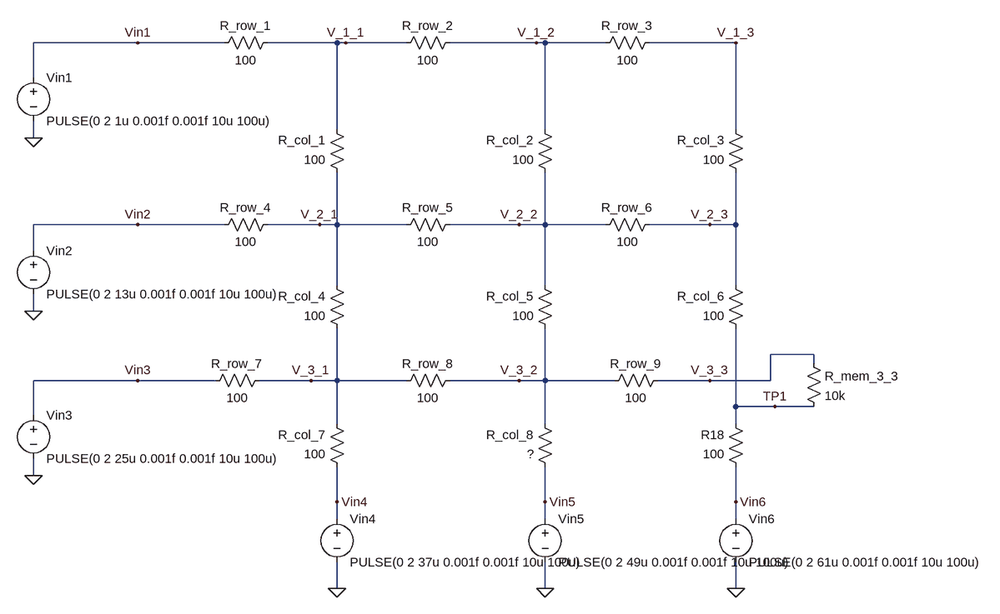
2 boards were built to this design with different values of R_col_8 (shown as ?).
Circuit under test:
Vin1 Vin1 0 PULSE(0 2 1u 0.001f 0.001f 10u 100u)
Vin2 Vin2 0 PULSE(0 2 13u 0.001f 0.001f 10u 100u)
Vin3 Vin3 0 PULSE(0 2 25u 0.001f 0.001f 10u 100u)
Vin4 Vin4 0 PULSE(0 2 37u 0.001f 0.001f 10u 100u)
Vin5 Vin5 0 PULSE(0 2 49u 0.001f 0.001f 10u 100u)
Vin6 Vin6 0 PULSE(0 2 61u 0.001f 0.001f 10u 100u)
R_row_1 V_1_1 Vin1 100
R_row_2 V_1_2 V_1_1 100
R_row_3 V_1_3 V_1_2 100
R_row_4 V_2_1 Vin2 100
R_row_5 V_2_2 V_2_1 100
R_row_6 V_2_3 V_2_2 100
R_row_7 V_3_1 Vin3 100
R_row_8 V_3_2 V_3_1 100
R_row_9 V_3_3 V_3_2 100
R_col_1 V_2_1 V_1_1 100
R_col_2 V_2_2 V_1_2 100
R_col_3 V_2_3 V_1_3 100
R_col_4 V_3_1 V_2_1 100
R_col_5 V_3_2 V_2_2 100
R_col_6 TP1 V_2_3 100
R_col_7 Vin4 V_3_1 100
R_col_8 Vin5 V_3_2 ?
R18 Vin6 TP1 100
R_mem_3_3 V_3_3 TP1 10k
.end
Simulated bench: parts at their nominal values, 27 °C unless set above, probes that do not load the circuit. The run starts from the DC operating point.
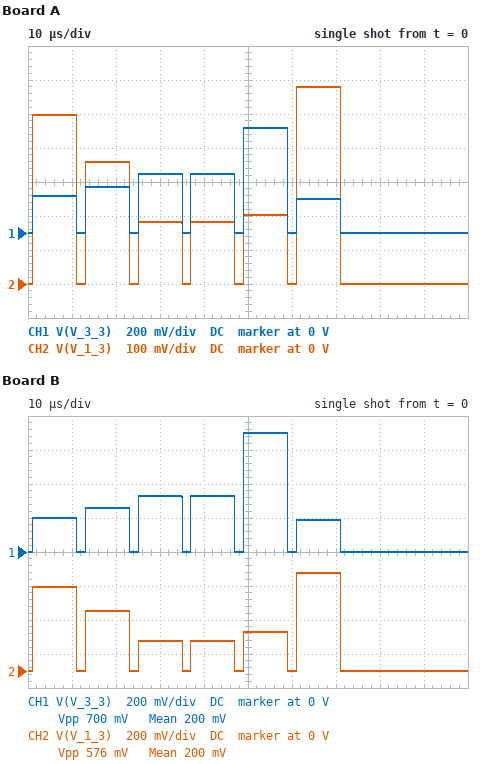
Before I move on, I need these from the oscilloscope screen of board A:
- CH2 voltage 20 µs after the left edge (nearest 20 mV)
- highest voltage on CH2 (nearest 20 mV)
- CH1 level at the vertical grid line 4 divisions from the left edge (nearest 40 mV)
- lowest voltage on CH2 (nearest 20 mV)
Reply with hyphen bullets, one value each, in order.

- 360 mV
- 580 mV
- 360 mV
- 0 V
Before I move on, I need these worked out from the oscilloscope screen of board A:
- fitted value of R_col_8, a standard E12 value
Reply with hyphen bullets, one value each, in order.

- 180 Ω
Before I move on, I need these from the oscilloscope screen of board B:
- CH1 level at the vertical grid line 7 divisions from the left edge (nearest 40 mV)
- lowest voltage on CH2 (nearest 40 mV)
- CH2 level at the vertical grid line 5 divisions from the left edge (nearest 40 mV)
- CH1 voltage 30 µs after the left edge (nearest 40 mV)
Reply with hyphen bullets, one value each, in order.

- 200 mV
- 0 V
- 240 mV
- 320 mV
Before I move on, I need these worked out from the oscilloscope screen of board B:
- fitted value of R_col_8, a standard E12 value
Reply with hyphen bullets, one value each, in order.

- 150 Ω
